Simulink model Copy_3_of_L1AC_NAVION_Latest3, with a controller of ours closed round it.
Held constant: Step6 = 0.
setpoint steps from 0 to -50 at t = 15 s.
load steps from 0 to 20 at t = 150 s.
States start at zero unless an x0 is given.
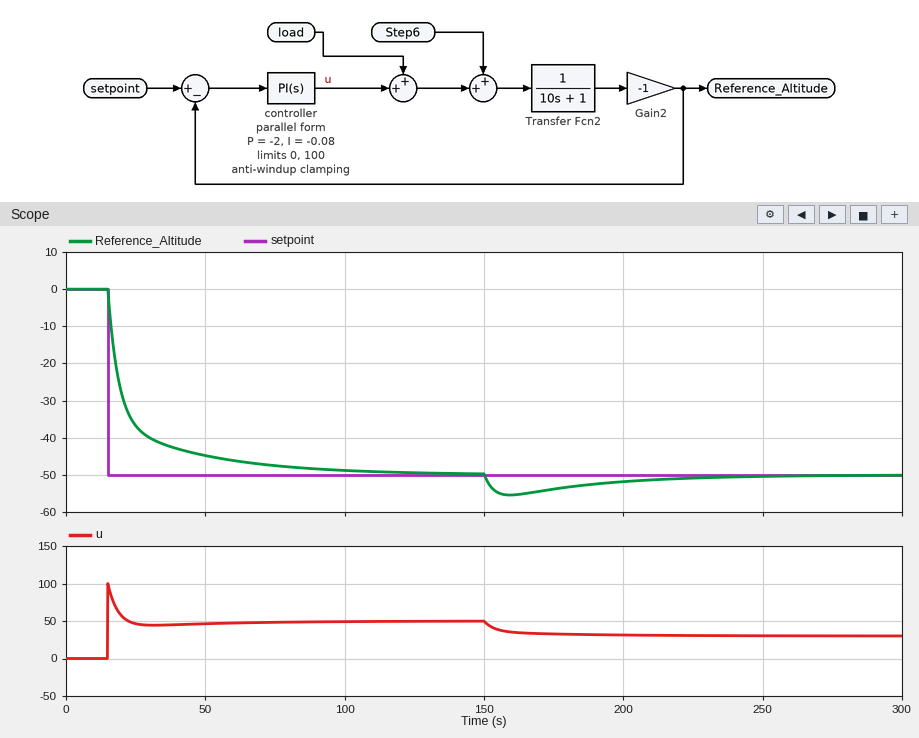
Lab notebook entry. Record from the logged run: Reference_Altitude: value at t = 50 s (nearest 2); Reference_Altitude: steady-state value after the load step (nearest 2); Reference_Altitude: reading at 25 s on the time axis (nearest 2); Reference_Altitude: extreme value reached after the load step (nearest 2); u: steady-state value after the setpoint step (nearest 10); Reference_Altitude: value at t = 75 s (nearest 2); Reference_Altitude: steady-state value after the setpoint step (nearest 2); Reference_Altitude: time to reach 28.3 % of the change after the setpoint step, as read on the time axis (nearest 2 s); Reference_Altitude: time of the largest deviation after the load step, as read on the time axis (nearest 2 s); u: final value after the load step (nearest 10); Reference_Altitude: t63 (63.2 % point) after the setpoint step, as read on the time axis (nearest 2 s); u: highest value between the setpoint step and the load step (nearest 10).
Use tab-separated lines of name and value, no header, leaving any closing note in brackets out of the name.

Reference_Altitude: value at t = 50 s	-44
Reference_Altitude: steady-state value after the load step	-50
Reference_Altitude: reading at 25 s on the time axis	-36
Reference_Altitude: extreme value reached after the load step	-56
u: steady-state value after the setpoint step	50
Reference_Altitude: value at t = 75 s	-48
Reference_Altitude: steady-state value after the setpoint step	-50
Reference_Altitude: time to reach 28.3 % of the change after the setpoint step, as read on the time axis	16 s
Reference_Altitude: time of the largest deviation after the load step, as read on the time axis	160 s
u: final value after the load step	30
Reference_Altitude: t63 (63.2 % point) after the setpoint step, as read on the time axis	22 s
u: highest value between the setpoint step and the load step	100
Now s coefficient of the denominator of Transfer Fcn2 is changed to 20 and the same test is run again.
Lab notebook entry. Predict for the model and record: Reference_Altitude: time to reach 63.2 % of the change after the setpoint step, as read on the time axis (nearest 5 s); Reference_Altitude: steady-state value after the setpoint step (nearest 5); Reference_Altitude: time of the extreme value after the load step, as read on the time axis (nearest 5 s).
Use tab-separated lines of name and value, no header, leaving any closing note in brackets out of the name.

Reference_Altitude: time to reach 63.2 % of the change after the setpoint step, as read on the time axis	25 s
Reference_Altitude: steady-state value after the setpoint step	-50
Reference_Altitude: time of the extreme value after the load step, as read on the time axis	165 s
